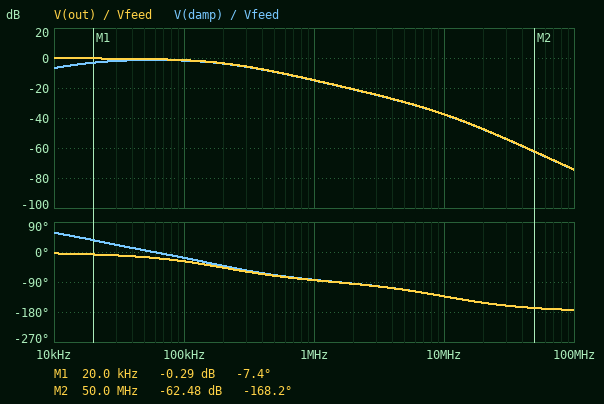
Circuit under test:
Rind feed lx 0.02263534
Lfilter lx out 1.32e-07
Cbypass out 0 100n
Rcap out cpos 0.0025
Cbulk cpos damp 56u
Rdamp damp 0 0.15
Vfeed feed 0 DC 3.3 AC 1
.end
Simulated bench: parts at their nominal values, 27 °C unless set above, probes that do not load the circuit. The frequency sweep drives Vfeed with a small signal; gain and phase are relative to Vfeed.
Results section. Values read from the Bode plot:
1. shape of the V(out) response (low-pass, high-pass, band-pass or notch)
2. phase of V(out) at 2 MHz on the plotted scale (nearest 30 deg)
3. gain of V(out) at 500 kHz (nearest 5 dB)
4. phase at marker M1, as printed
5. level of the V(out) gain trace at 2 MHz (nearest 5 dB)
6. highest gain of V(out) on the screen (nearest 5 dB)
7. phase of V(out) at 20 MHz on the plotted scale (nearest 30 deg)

low-pass
-90 deg
-10 dB
-7.4 deg
-20 dB
0 dB
-150 deg
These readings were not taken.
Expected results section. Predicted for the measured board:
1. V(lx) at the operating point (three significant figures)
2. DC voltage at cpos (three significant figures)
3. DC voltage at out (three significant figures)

3.30 V
3.30 V
3.30 V
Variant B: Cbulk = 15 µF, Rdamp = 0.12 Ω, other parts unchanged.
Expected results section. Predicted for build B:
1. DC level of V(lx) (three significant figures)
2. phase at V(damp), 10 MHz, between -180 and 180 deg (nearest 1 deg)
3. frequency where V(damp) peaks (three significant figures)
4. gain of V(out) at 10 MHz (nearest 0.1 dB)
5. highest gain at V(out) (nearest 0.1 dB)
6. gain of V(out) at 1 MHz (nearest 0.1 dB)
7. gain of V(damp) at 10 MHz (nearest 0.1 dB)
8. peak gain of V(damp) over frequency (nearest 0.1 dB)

3.30 V
-127 deg
113 kHz
-38.6 dB
1.1 dB
-16.6 dB
-38.8 dB
-1.6 dB
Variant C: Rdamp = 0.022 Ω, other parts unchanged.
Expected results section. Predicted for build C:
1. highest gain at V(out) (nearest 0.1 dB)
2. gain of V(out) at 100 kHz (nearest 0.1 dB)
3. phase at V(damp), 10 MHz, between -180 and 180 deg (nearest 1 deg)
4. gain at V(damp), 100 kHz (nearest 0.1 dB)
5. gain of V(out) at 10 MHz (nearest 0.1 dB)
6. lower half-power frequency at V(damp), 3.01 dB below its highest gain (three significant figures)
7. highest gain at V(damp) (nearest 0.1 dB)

2.0 dB
-5.7 dB
-98 deg
-10.3 dB
-50.7 dB
36.6 kHz
-6.6 dB
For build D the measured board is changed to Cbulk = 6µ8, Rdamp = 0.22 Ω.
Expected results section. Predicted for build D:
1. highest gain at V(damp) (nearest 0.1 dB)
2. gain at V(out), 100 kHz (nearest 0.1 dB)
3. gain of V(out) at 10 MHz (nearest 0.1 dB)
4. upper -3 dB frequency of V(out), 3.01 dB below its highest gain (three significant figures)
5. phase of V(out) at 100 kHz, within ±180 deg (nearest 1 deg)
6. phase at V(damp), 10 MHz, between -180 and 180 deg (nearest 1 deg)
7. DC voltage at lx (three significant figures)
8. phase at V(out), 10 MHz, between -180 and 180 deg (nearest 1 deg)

-0.8 dB
1.0 dB
-36.1 dB
301 kHz
-15 deg
-143 deg
3.30 V
-144 deg
